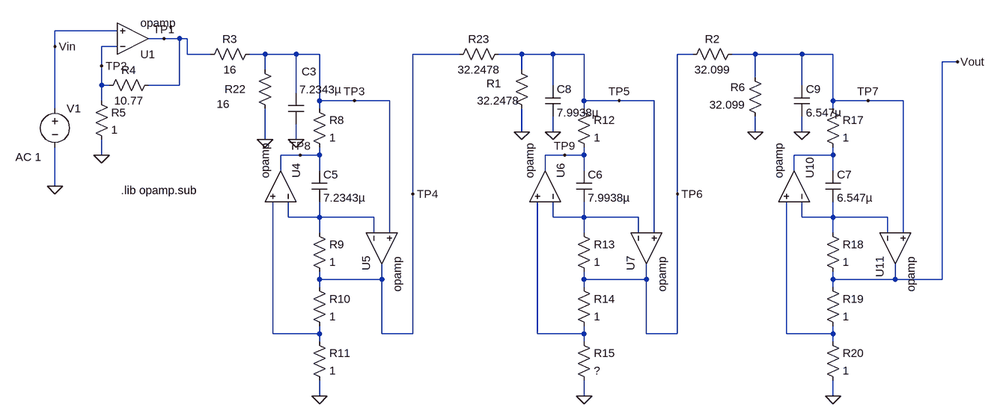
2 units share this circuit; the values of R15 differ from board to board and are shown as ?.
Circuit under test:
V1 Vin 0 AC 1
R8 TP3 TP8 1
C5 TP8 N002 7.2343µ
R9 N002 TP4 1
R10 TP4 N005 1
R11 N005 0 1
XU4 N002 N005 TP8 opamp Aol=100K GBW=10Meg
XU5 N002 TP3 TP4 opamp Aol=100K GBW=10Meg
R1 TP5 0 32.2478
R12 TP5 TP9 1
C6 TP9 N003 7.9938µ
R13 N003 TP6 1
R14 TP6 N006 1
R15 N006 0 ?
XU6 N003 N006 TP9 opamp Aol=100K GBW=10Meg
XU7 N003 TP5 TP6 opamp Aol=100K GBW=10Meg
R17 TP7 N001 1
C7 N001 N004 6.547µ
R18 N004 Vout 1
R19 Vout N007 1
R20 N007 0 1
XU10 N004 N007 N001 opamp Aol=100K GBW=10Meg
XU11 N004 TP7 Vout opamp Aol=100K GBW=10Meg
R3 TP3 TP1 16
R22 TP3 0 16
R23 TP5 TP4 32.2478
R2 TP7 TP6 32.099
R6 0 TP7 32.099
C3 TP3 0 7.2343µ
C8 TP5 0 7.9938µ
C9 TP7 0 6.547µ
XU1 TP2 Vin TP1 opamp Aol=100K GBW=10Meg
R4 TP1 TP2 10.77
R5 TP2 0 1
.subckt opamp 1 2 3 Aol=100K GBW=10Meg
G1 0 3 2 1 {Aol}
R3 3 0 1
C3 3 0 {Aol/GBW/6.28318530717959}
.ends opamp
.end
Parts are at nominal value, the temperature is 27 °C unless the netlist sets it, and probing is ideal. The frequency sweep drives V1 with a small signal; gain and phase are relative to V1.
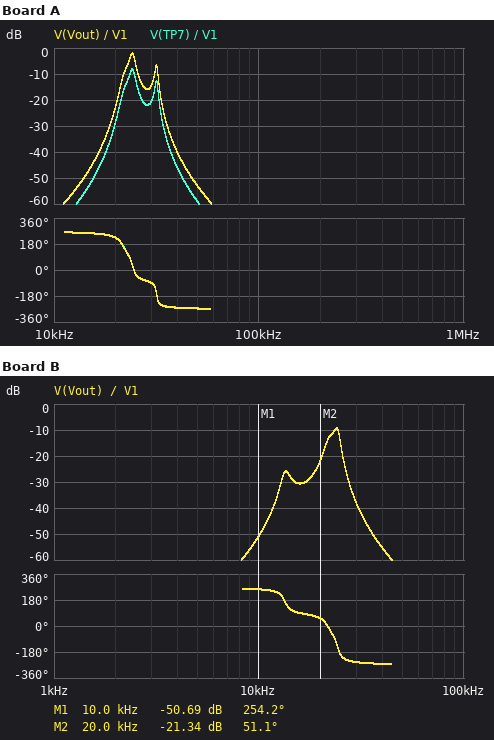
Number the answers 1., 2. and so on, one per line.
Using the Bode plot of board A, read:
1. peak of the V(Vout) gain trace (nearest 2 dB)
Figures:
1. -2 dB
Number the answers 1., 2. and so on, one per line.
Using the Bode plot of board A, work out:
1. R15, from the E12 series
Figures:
1. 0.39 Ω
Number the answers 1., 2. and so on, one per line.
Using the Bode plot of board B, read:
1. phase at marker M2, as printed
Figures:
1. 51.1 deg
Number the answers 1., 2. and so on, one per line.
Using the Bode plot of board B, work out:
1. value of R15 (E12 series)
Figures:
1. 2.2 Ω
